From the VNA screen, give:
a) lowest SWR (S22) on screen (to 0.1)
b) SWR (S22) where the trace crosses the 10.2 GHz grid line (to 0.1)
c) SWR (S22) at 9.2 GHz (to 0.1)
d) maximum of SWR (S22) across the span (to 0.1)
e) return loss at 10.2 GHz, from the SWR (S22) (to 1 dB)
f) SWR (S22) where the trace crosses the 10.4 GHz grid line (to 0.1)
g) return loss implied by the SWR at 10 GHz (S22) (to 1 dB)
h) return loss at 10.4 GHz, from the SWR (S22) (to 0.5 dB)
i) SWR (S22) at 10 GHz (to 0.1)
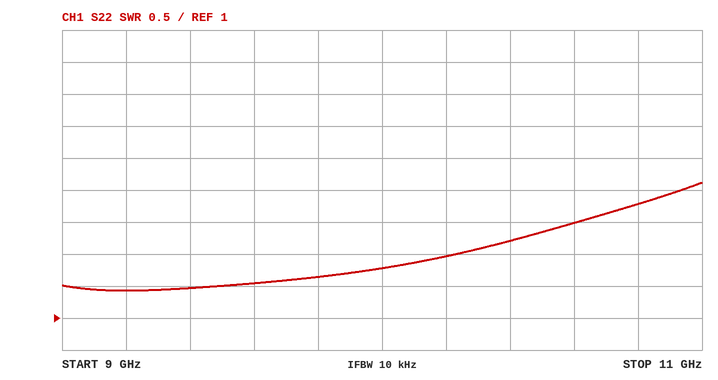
1.4
2.0
1.4
3.1
10 dB
2.2
11 dB
8.5 dB
1.8
